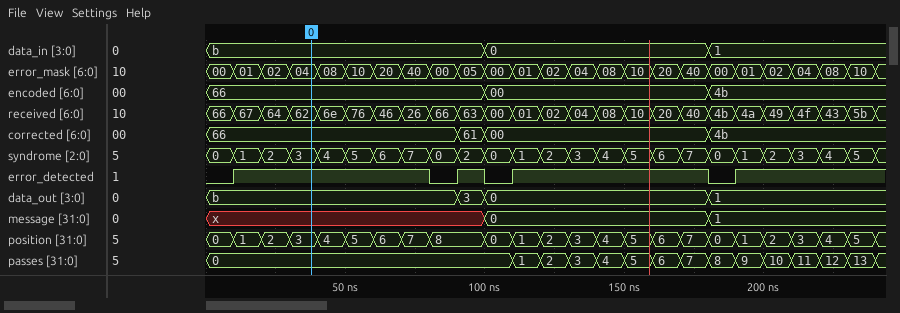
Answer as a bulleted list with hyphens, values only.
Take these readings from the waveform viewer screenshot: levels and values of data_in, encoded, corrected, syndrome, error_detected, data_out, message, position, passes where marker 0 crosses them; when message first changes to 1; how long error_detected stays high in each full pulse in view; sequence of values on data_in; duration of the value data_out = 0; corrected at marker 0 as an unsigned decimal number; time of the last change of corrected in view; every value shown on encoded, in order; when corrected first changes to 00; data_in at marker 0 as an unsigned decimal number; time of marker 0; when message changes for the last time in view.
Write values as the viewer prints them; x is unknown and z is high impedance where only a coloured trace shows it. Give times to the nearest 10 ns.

- data_in=b, encoded=66, corrected=66, syndrome=3, error_detected=1, data_out=b, message=x, position=3, passes=0
- 180 ns
- 70 ns, 10 ns, 70 ns
- b, 0, 1
- 80 ns
- 102
- 180 ns
- 66, 00, 4b
- 100 ns
- 11
- 40 ns
- 180 ns
